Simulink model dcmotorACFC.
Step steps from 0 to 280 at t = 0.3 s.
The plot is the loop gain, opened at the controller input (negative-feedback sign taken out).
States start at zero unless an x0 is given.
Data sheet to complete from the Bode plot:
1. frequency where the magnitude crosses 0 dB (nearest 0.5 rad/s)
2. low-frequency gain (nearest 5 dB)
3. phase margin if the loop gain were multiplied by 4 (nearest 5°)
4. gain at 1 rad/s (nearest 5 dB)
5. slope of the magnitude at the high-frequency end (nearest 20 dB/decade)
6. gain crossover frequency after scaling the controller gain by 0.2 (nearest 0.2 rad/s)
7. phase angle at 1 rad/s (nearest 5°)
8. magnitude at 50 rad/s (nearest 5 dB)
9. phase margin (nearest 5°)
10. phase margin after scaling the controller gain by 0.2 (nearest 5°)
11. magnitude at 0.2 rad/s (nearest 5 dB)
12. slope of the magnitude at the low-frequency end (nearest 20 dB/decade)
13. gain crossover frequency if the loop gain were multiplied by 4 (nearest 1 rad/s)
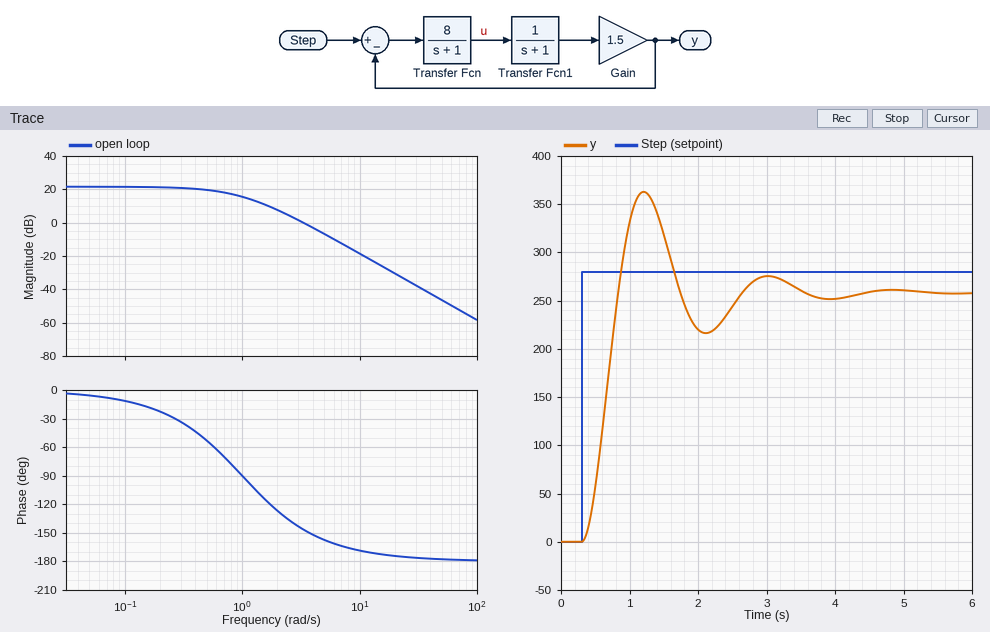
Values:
3.5 rad/s
20 dB
15°
15 dB
-40 dB/decade
1.2 rad/s
-90°
-45 dB
35°
80°
20 dB
0 dB/decade
7 rad/s
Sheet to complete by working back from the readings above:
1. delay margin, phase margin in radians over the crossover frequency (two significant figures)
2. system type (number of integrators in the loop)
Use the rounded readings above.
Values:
0.17 s
0
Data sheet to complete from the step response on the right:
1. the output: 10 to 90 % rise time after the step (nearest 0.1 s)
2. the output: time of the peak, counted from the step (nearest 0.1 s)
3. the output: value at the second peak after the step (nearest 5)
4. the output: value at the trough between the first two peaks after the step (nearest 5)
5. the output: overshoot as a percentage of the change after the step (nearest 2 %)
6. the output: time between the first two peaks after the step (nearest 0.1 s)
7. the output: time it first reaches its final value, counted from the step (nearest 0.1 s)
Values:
0.4 s
0.9 s
275
215
40 %
1.8 s
0.5 s
